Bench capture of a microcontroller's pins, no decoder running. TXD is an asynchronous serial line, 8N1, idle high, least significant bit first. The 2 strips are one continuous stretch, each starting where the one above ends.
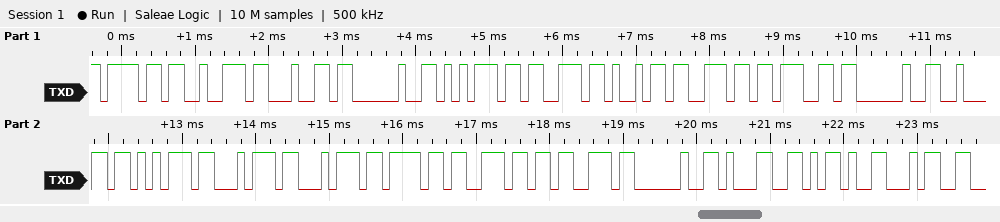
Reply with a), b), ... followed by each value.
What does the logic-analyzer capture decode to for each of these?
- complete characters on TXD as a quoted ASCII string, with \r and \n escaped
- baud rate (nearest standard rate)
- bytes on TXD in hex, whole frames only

a) "ord using buttons 1-4"
b) 9600 baud
c) 6F 72 64 20 75 73 69 6E 67 20 62 75 74 74 6F 6E 73 20 31 2D 34
